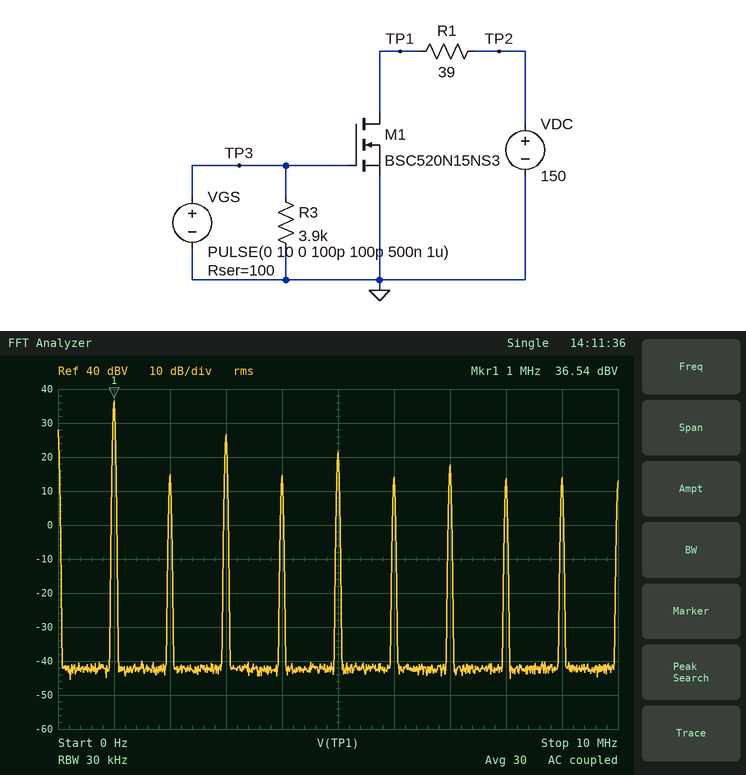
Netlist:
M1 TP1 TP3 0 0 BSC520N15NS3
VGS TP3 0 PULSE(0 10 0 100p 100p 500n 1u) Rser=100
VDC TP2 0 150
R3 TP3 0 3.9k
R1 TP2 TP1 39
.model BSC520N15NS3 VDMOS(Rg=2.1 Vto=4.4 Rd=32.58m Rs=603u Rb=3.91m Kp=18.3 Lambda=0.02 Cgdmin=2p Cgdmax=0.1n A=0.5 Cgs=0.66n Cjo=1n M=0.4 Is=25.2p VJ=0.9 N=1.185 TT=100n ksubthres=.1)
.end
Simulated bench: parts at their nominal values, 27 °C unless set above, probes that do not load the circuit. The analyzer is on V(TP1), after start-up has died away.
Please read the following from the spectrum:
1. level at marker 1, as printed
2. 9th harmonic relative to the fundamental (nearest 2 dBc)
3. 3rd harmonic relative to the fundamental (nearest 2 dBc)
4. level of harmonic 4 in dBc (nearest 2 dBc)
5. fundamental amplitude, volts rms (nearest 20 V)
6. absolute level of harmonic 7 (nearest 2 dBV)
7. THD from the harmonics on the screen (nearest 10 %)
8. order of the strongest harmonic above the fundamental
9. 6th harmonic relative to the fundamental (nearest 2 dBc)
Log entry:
36.54 dBV
-22 dBc
-10 dBc
-22 dBc
60 V
18 dBV
40 %
3
-22 dBc
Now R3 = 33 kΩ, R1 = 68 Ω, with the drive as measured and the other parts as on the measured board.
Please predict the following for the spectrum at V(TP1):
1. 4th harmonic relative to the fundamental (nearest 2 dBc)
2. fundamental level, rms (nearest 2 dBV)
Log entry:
-20 dBc
36 dBV
